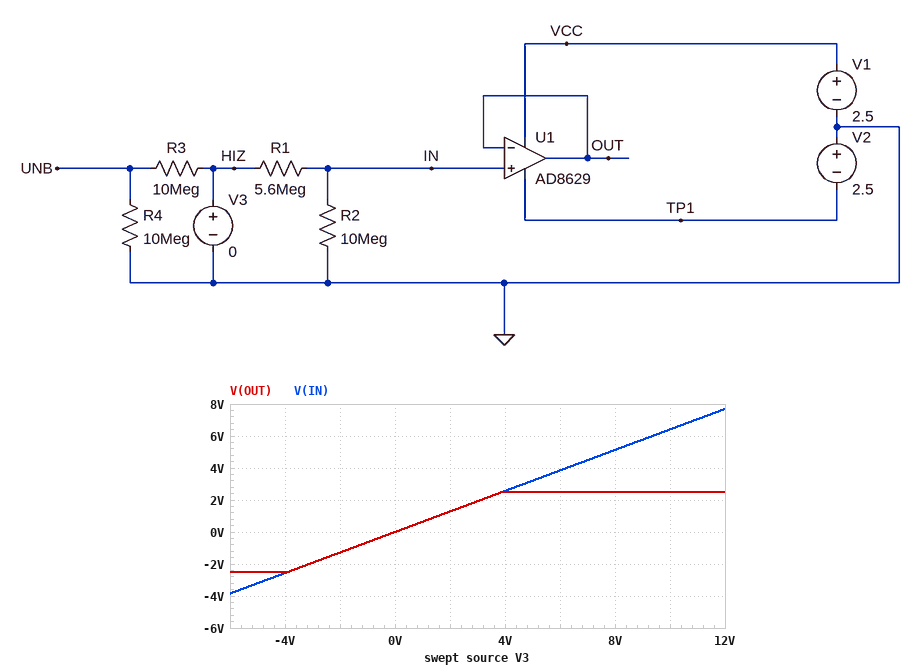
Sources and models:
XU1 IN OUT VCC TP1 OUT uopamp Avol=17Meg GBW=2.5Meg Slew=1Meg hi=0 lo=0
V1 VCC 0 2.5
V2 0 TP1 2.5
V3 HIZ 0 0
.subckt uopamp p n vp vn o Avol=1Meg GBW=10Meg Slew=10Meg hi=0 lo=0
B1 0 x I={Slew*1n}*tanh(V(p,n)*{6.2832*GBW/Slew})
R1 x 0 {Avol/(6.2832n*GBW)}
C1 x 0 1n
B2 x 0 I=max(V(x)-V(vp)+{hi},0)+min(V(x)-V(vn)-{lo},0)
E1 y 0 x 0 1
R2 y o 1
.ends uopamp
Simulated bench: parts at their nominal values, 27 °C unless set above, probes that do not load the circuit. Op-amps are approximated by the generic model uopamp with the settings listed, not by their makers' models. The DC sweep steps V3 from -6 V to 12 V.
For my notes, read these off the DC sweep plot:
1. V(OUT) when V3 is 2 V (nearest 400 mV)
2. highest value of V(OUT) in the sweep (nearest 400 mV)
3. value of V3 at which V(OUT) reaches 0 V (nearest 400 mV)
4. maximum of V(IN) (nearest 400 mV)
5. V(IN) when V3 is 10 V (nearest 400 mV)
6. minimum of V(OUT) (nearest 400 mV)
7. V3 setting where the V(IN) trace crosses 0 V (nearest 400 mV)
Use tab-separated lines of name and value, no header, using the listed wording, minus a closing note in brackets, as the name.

V(OUT) when V3 is 2 V	1.2 V
highest value of V(OUT) in the sweep	2.4 V
value of V3 at which V(OUT) reaches 0 V	0 V
maximum of V(IN)	7.6 V
V(IN) when V3 is 10 V	6.4 V
minimum of V(OUT)	-2.4 V
V3 setting where the V(IN) trace crosses 0 V	0 V
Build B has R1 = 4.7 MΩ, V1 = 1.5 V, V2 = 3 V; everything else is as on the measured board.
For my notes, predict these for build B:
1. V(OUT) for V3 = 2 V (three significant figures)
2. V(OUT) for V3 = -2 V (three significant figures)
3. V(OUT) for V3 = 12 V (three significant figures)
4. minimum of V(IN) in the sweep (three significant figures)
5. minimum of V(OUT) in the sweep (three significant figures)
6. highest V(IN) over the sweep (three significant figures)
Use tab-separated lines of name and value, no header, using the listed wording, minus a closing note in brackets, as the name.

V(OUT) for V3 = 2 V	1.36 V
V(OUT) for V3 = -2 V	-1.36 V
V(OUT) for V3 = 12 V	1.50 V
minimum of V(IN) in the sweep	-4.08 V
minimum of V(OUT) in the sweep	-3.00 V
highest V(IN) over the sweep	8.16 V
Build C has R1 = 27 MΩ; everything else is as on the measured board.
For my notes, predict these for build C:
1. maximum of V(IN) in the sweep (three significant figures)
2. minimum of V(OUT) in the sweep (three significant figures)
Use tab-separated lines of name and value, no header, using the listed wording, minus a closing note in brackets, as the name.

maximum of V(IN) in the sweep	3.24 V
minimum of V(OUT) in the sweep	-1.62 V
